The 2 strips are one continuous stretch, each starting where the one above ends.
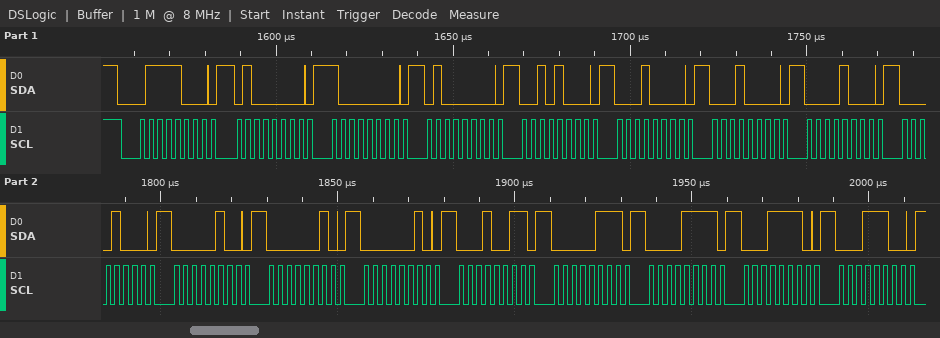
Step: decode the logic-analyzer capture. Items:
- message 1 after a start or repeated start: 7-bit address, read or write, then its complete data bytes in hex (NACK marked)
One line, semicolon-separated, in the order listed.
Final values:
0x3C write: 40 80 40 28 10 10 08 08 04 02 02 13 07 0F 1E 1C
